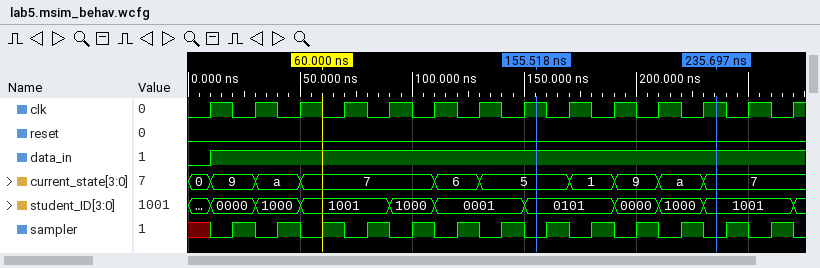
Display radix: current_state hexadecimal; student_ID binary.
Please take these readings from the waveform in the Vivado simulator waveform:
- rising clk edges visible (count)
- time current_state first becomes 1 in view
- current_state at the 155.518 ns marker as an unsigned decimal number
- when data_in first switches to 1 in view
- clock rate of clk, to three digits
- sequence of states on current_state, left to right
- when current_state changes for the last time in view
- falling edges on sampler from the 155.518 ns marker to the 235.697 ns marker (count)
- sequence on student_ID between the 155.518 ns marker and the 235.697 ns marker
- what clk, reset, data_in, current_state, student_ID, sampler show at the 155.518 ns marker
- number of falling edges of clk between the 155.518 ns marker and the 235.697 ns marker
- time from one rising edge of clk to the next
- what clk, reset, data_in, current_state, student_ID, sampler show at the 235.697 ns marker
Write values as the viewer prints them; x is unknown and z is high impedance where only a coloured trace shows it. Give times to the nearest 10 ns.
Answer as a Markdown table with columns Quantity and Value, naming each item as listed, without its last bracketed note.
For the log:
| Quantity | Value |
|---|---|
| rising clk edges visible | 14 |
| time current_state first becomes 1 in view | 170 ns |
| current_state at the 155.518 ns marker as an unsigned decimal number | 5 |
| when data_in first switches to 1 in view | 10 ns |
| clock rate of clk, to three digits | 50.0 MHz |
| sequence of states on current_state, left to right | 0, 9, a, 7, 6, 5, 1, 9, a, 7 |
| when current_state changes for the last time in view | 230 ns |
| falling edges on sampler from the 155.518 ns marker to the 235.697 ns marker | 4 |
| sequence on student_ID between the 155.518 ns marker and the 235.697 ns marker | 0101, 0000, 1000, 1001 |
| what clk, reset, data_in, current_state, student_ID, sampler show at the 155.518 ns marker | clk=1, reset=0, data_in=1, current_state=5, student_ID=0101, sampler=0 |
| number of falling edges of clk between the 155.518 ns marker and the 235.697 ns marker | 4 |
| time from one rising edge of clk to the next | 20 ns |
| what clk, reset, data_in, current_state, student_ID, sampler show at the 235.697 ns marker | clk=1, reset=0, data_in=1, current_state=7, student_ID=1001, sampler=0 |
